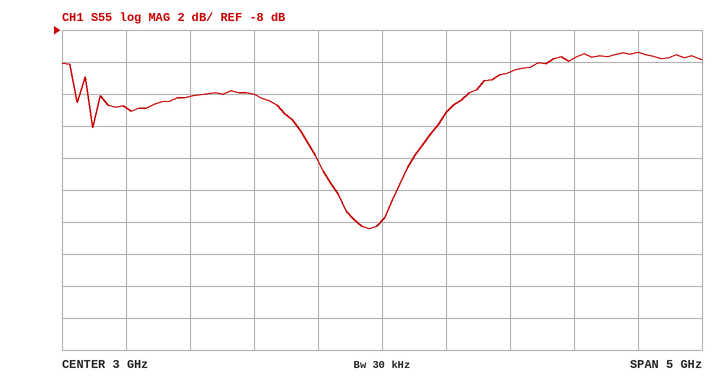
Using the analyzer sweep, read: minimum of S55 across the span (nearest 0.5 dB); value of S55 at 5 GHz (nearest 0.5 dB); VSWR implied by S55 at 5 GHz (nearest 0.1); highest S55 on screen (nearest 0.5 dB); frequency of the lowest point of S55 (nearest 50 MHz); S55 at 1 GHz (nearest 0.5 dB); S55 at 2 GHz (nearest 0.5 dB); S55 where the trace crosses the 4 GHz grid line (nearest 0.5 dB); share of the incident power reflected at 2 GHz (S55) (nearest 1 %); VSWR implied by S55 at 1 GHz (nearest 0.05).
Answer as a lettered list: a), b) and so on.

a) -20.5 dB
b) -9.5 dB
c) 2.0
d) -9.5 dB
e) 2.90 GHz
f) -13.0 dB
g) -12.0 dB
h) -10.5 dB
i) 6 %
j) 1.60
